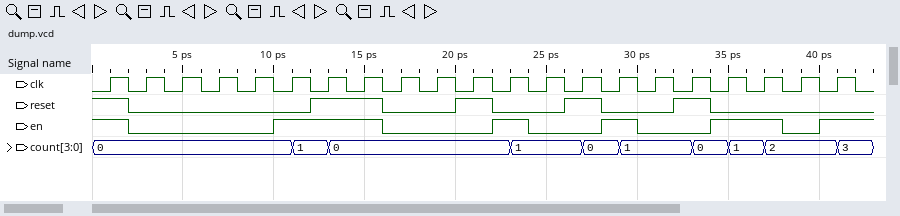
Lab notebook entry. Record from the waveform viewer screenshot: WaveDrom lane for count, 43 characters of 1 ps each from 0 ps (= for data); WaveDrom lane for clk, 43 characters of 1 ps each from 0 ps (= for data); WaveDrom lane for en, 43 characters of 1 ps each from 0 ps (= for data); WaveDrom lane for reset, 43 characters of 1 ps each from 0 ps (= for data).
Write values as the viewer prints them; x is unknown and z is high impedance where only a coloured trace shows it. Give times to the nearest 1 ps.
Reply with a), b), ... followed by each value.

a) {name: 'count', wave: '=..........=.=.........=...=.=...=.=.=...=.', data: '0 1 0 1 0 1 0 1 2 3'}
b) {name: 'clk', wave: '0101010101010101010101010101010101010101010'}
c) {name: 'en', wave: '1.0.......1.....0.....1.0...1.0...1...0.1..'}
d) {name: 'reset', wave: '1.0.........1...0...1.0...1.0...1.0........'}
